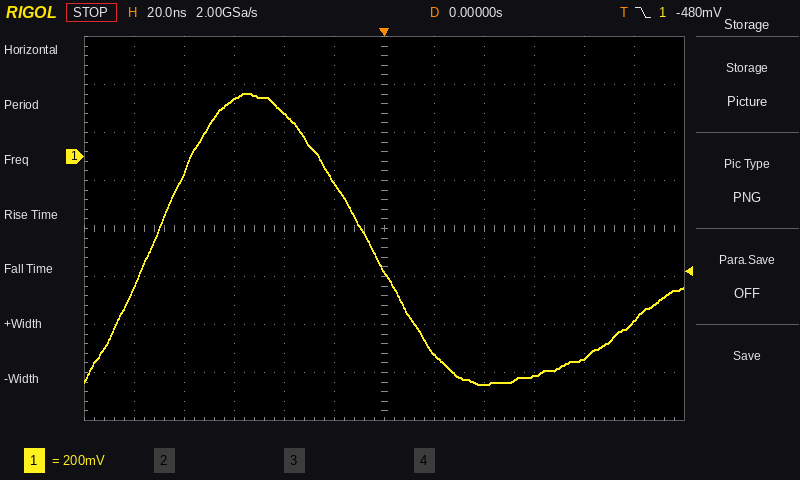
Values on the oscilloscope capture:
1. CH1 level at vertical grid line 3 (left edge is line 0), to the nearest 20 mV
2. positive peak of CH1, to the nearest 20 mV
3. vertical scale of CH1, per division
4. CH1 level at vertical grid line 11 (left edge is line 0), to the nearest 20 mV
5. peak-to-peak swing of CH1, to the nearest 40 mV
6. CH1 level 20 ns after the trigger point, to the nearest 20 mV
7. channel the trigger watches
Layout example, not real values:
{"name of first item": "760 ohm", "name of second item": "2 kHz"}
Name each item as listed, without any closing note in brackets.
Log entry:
{"CH1 level at vertical grid line 3 (left edge is line 0), to the nearest 20 mV": "240 mV", "positive peak of CH1, to the nearest 20 mV": "260 mV", "vertical scale of CH1, per division": "200 mV", "CH1 level at vertical grid line 11 (left edge is line 0), to the nearest 20 mV": "-680 mV", "peak-to-peak swing of CH1, to the nearest 40 mV": "1.20 V", "CH1 level 20 ns after the trigger point, to the nearest 20 mV": "-820 mV", "channel the trigger watches": "CH1"}
